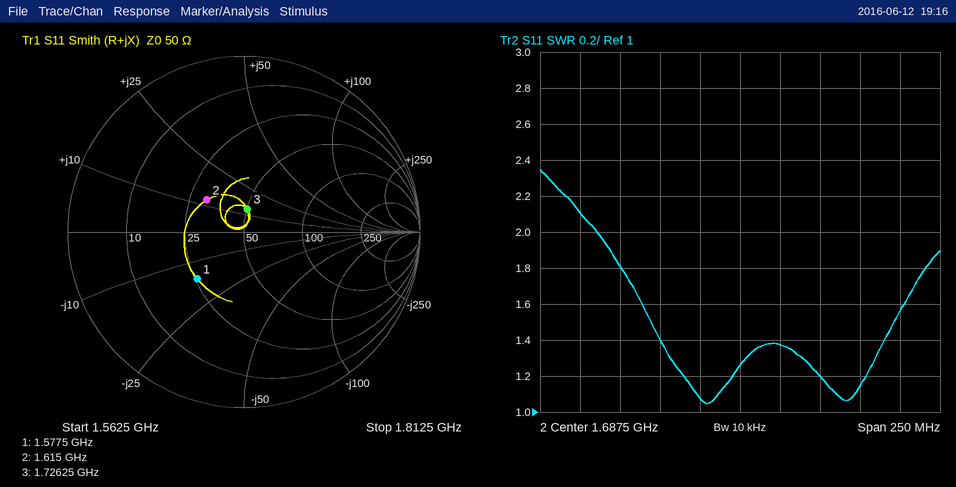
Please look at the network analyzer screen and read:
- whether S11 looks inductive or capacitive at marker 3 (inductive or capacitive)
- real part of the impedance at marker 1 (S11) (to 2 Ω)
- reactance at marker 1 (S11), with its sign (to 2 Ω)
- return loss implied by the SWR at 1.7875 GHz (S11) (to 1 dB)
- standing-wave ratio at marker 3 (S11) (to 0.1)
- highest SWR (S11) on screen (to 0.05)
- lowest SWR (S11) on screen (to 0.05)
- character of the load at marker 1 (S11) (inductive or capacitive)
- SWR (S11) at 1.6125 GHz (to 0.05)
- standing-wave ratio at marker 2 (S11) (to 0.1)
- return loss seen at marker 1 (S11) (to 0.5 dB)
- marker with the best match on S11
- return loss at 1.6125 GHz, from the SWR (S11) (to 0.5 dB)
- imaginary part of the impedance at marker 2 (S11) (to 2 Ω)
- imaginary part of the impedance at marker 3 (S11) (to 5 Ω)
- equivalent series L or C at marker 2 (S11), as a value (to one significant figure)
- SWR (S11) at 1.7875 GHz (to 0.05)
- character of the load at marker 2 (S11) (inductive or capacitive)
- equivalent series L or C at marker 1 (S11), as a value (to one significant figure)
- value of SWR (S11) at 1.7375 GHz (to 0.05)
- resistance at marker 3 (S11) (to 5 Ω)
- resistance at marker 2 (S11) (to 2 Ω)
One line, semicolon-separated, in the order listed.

inductive; 26 Ω; -16 Ω; 13 dB; 1.3; 2.35; 1.05; capacitive; 1.80; 1.8; 8.5 dB; marker 3; 11.0 dB; +12 Ω; +15 Ω; 1 nH; 1.55; inductive; 6 pF; 1.20; 50 Ω; 30 Ω
